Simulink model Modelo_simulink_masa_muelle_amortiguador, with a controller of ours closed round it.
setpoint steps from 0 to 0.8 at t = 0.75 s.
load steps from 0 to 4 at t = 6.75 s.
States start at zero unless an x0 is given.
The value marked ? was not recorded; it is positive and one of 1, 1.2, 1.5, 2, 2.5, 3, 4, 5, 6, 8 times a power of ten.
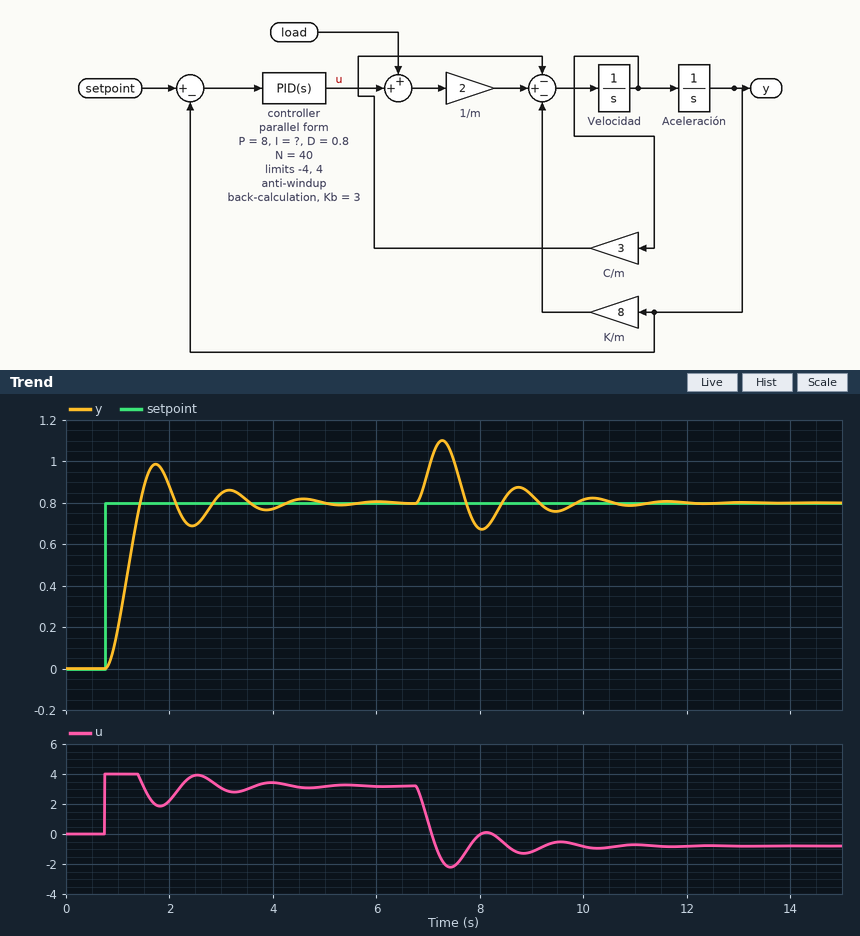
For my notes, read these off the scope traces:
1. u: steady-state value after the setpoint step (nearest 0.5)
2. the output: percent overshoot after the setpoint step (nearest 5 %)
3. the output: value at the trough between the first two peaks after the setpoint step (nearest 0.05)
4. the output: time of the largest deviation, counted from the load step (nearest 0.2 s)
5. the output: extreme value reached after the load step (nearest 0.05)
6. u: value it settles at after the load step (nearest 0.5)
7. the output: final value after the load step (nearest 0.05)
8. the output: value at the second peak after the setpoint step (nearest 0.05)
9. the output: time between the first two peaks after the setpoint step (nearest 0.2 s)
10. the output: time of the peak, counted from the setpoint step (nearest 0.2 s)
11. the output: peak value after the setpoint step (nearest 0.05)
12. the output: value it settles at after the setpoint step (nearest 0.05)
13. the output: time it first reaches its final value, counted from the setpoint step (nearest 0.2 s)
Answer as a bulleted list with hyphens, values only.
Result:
- 3.0
- 25 %
- 0.70
- 0.6 s
- 1.10
- -1.0
- 0.80
- 0.85
- 1.4 s
- 1.0 s
- 1.00
- 0.80
- 0.6 s
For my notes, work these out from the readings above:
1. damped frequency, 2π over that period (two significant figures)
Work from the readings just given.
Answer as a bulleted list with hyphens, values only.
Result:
- 4.5 rad/s
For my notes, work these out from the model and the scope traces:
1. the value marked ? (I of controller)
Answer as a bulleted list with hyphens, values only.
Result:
- 30
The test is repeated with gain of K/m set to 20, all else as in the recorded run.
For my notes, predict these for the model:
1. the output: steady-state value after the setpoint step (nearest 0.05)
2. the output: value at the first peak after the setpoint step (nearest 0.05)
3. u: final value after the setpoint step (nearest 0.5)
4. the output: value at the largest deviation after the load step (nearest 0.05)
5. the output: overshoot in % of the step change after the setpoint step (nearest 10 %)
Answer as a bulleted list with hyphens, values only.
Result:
- 0.40
- 0.55
- 4.0
- 0.90
- 30 %
